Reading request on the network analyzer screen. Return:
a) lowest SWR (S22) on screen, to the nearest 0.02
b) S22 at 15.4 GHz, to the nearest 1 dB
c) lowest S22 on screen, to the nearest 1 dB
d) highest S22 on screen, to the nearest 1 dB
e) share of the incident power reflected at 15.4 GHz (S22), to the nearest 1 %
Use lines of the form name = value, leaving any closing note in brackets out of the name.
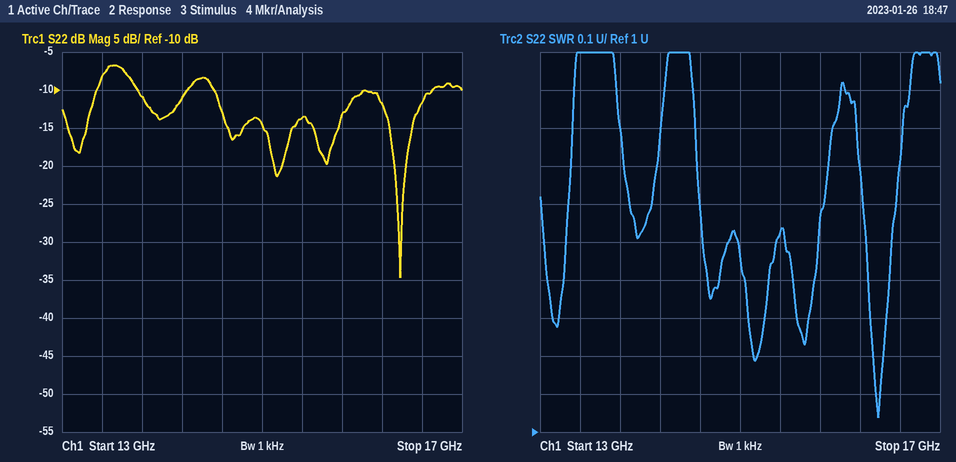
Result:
lowest SWR (S22) on screen, to the nearest 0.02 = 1.04
S22 at 15.4 GHz, to the nearest 1 dB = -14 dB
lowest S22 on screen, to the nearest 1 dB = -35 dB
highest S22 on screen, to the nearest 1 dB = -7 dB
share of the incident power reflected at 15.4 GHz (S22), to the nearest 1 % = 4 %
